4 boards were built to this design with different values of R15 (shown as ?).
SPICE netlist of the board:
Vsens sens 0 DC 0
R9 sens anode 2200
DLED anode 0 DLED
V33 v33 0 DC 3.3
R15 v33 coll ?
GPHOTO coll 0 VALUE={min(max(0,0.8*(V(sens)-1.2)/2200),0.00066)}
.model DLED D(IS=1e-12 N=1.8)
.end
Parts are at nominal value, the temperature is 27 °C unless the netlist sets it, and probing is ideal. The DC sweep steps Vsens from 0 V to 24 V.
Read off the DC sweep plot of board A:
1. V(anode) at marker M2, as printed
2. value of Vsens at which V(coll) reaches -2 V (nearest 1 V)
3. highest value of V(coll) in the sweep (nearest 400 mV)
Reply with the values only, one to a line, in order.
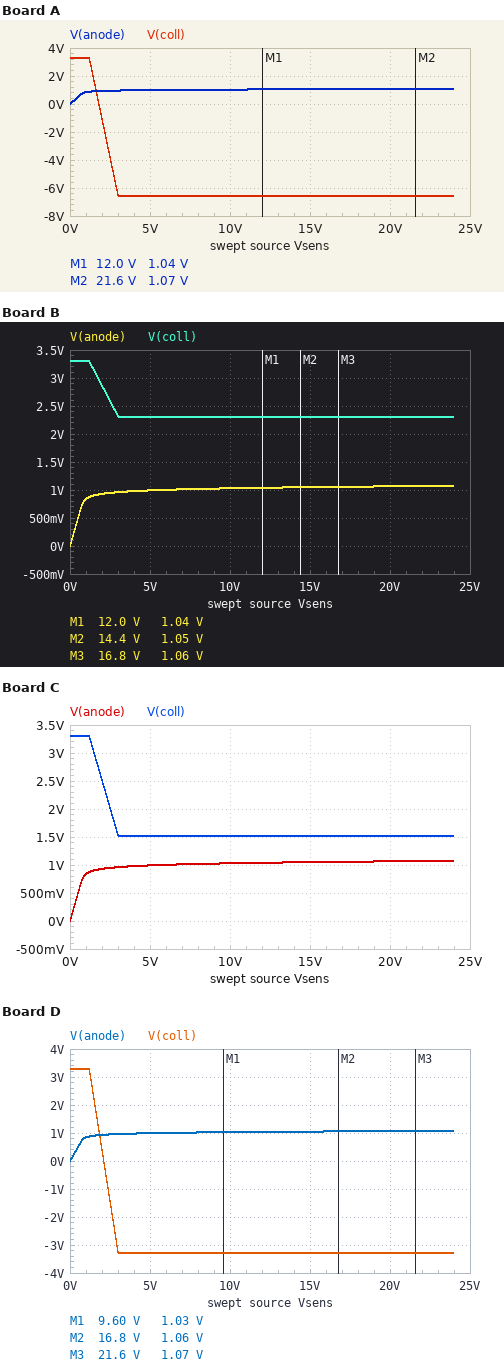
1.07 V
2 V
3.2 V
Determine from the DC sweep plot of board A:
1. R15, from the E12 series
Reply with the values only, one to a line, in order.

15 kΩ
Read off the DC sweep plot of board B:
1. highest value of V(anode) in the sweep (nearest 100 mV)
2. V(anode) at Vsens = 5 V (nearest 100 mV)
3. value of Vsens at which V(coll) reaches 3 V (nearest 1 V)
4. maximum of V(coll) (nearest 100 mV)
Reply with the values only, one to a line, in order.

1.1 V
1.0 V
2 V
3.3 V
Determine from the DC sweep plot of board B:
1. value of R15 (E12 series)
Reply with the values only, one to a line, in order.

1.5 kΩ
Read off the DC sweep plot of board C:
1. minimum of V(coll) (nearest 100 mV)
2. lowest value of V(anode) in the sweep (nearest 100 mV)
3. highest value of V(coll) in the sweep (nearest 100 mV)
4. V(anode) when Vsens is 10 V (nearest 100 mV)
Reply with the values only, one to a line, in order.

1.5 V
0 V
3.3 V
1.0 V
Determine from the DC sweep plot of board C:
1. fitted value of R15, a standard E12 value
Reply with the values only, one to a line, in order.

2.7 kΩ
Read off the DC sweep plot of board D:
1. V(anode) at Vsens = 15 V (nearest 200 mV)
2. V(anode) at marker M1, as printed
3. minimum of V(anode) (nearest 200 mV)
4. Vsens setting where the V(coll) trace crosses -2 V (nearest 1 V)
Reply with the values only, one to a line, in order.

1.0 V
1.03 V
0 V
3 V
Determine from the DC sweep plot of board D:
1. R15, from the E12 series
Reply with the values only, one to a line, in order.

10 kΩ
